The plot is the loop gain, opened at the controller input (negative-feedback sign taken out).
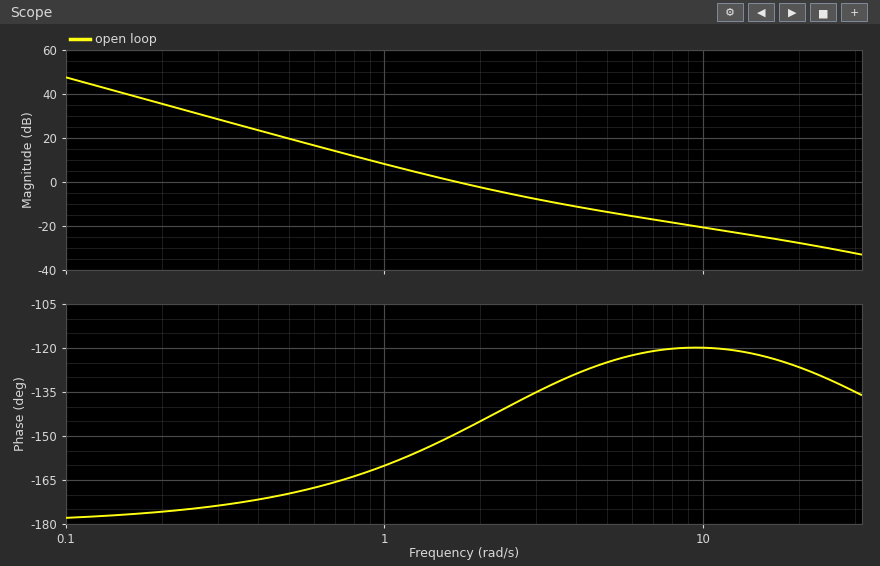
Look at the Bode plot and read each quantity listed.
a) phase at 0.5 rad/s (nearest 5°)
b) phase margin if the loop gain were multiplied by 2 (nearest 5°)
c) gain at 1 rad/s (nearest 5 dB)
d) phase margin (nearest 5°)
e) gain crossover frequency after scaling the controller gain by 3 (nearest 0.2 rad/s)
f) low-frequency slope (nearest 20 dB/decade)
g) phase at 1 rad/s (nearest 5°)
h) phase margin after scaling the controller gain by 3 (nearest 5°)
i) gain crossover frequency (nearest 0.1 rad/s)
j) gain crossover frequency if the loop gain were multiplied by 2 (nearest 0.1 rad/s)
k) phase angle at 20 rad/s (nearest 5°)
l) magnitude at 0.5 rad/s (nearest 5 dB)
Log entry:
-170°
40°
10 dB
30°
3.4 rad/s
-40 dB/decade
-160°
50°
1.7 rad/s
2.6 rad/s
-125°
20 dB
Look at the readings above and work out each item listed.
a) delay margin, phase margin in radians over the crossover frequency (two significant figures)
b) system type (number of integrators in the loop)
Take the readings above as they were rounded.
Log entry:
0.31 s
2
